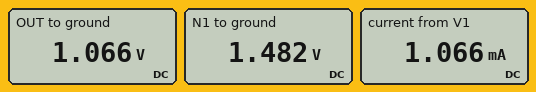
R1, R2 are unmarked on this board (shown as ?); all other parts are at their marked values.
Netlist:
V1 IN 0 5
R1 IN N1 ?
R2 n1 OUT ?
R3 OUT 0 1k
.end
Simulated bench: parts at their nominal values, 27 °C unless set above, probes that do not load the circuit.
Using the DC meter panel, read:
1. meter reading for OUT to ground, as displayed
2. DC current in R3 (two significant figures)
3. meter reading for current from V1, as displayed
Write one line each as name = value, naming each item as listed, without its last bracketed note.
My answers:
meter reading for OUT to ground, as displayed = 1.066 V
DC current in R3 = 1.1 mA
meter reading for current from V1, as displayed = 1.066 mA
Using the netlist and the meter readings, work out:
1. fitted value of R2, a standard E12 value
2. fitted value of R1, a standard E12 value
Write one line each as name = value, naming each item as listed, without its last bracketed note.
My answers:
fitted value of R2, a standard E12 value = 390 Ω
fitted value of R1, a standard E12 value = 3.3 kΩ
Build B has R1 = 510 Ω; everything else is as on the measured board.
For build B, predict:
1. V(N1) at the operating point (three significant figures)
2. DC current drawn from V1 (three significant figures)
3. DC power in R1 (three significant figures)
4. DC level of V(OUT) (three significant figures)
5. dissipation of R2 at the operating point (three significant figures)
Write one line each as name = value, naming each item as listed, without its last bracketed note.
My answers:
V(N1) at the operating point = 3.66 V
DC current drawn from V1 = 2.63 mA
DC power in R1 = 3.53 mW
DC level of V(OUT) = 2.63 V
dissipation of R2 at the operating point = 2.70 mW
